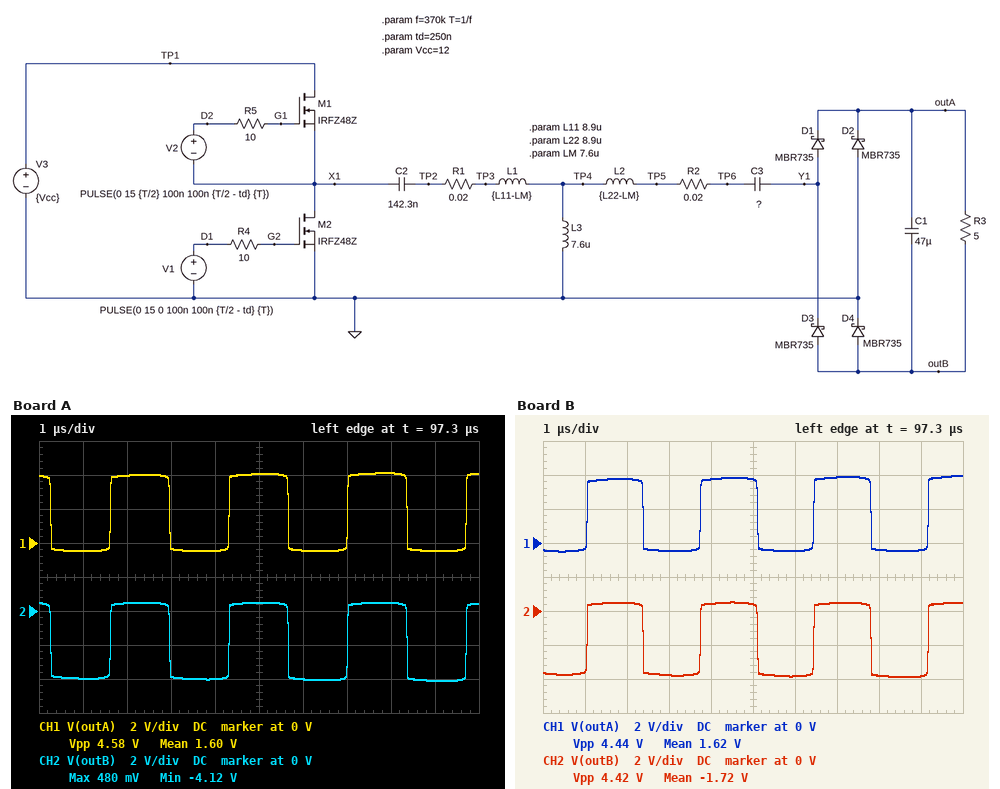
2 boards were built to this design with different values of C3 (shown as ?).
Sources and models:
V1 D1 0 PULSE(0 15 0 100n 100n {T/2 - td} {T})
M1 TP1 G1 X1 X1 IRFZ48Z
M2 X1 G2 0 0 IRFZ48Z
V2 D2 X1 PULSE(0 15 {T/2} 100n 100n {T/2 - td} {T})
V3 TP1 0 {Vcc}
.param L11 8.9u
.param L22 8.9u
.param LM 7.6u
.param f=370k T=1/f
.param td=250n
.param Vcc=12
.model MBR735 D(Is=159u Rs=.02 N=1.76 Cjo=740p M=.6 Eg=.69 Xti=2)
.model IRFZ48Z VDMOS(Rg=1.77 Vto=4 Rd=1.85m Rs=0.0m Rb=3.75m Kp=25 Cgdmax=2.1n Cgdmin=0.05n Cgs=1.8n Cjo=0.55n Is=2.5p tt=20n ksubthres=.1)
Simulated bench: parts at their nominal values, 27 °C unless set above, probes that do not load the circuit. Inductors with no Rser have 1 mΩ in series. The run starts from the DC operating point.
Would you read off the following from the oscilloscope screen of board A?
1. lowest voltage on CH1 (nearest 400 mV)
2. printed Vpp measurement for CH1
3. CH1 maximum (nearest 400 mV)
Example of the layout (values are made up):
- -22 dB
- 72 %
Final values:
- -400 mV
- 4.58 V
- 4.0 V
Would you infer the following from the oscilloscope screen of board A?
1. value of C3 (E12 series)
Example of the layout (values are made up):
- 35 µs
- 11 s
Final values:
- 390 nF
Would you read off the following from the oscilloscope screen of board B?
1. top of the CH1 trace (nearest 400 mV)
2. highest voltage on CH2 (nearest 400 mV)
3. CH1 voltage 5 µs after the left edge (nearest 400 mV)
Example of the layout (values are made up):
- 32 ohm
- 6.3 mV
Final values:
- 4.0 V
- 400 mV
- 3.6 V
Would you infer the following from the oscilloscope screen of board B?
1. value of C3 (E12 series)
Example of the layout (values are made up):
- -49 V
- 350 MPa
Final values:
- 82 nF
